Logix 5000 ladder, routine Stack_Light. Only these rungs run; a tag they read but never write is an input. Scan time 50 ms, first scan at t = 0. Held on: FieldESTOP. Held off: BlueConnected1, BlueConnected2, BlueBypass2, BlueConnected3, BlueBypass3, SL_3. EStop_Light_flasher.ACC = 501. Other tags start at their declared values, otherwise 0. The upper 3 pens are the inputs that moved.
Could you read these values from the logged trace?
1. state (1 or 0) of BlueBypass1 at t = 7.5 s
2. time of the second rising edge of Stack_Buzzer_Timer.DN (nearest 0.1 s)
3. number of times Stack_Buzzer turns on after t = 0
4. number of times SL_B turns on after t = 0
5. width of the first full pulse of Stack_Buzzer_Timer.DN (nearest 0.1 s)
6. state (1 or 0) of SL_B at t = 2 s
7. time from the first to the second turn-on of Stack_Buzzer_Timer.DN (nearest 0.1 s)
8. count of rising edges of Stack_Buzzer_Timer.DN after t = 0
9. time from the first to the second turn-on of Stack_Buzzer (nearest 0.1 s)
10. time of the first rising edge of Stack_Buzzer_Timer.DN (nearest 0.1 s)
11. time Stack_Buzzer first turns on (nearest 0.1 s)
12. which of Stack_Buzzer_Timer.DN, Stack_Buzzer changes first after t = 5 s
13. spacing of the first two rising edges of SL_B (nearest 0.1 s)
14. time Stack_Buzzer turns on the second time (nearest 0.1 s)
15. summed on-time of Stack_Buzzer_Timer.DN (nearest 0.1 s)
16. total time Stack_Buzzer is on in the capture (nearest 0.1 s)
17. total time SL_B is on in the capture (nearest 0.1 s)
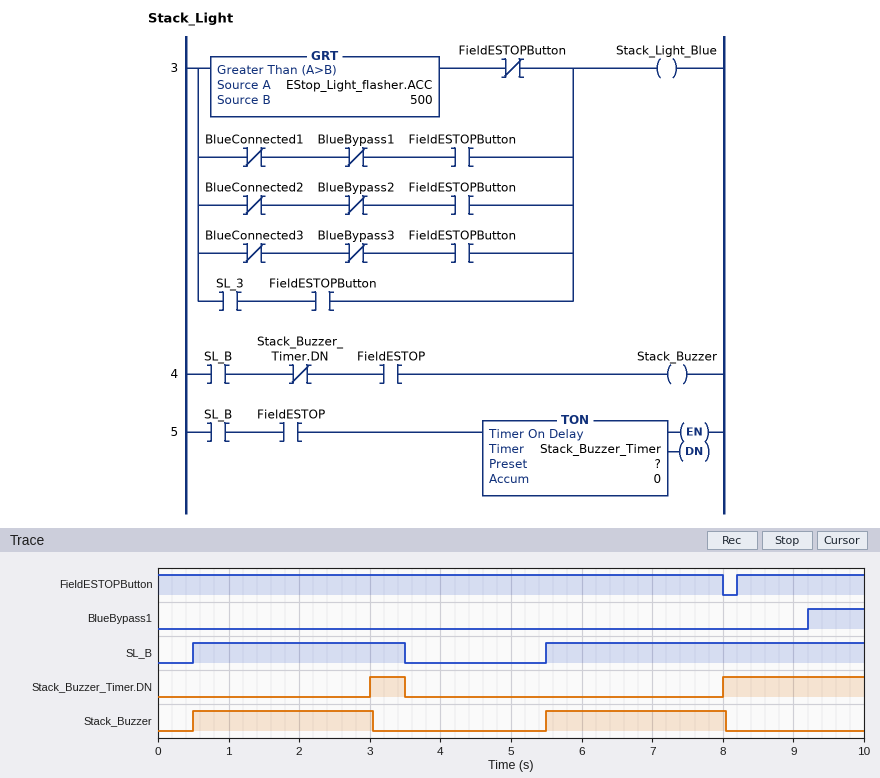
0
8.0 s
2
2
0.5 s
1
5.0 s
2
5.0 s
3.0 s
0.5 s
Stack_Buzzer
5.0 s
5.5 s
2.5 s
5.1 s
7.5 s
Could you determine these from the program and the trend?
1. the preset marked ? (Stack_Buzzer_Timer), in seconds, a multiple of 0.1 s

2.5 s
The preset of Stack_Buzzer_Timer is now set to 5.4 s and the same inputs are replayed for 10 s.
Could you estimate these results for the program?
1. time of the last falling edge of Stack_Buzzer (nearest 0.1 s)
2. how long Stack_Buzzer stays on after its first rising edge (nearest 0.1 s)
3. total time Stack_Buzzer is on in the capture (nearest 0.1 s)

3.5 s
3.0 s
7.5 s
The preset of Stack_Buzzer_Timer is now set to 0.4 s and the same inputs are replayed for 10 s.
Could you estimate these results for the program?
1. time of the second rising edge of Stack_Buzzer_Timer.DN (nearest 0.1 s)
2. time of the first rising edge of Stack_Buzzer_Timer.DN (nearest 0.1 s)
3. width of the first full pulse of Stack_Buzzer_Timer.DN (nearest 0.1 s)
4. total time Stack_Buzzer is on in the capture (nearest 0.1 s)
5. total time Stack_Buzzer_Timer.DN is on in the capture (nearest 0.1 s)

5.9 s
0.9 s
2.6 s
0.9 s
6.7 s
